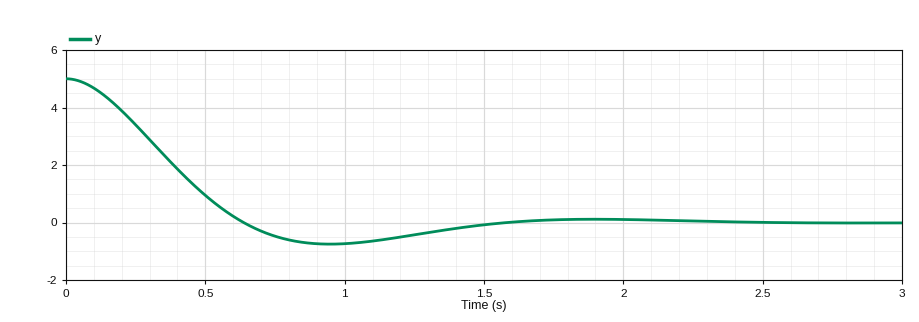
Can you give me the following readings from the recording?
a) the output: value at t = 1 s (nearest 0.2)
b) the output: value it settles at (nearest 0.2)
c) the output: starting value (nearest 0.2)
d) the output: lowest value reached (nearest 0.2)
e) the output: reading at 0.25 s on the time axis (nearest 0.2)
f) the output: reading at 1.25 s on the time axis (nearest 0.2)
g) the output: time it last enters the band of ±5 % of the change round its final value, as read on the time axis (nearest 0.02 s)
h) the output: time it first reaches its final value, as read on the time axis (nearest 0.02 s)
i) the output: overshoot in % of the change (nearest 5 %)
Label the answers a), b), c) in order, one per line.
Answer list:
a) -0.8
b) 0.0
c) 5.0
d) -0.8
e) 3.4
f) -0.4
g) 1.36 s
h) 0.64 s
i) 15 %
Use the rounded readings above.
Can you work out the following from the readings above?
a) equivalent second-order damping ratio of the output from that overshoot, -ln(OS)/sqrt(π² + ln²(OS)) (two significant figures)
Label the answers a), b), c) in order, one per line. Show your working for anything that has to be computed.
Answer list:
a) ln(0.15) = -1.897; 1.897 / sqrt(9.870 + 3.599) = 0.52
